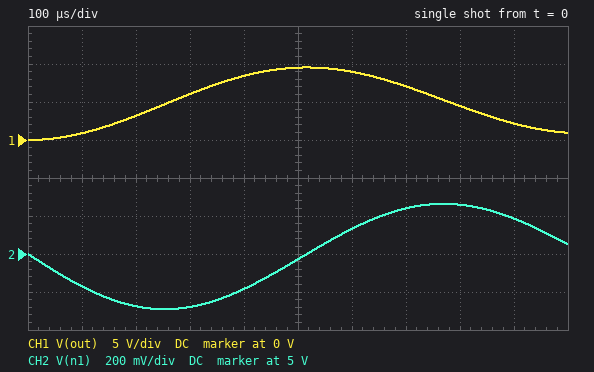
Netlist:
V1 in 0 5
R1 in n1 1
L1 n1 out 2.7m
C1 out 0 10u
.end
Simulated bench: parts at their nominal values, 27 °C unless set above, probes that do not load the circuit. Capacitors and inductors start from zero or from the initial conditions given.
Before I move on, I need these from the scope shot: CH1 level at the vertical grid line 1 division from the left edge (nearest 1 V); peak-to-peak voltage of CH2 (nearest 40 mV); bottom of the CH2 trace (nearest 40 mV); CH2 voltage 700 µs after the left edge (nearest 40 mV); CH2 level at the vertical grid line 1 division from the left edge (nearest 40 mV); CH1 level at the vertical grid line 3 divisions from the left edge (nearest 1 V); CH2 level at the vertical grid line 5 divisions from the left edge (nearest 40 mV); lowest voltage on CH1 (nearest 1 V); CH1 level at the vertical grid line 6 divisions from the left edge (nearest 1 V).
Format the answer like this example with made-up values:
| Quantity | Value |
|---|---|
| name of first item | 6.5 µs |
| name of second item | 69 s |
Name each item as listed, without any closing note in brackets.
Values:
| Quantity | Value |
|---|---|
| CH1 level at the vertical grid line 1 division from the left edge | 1 V |
| peak-to-peak voltage of CH2 | 560 mV |
| bottom of the CH2 trace | 4.72 V |
| CH2 voltage 700 µs after the left edge | 5.24 V |
| CH2 level at the vertical grid line 1 division from the left edge | 4.84 V |
| CH1 level at the vertical grid line 3 divisions from the left edge | 6 V |
| CH2 level at the vertical grid line 5 divisions from the left edge | 4.96 V |
| lowest voltage on CH1 | 0 V |
| CH1 level at the vertical grid line 6 divisions from the left edge | 9 V |
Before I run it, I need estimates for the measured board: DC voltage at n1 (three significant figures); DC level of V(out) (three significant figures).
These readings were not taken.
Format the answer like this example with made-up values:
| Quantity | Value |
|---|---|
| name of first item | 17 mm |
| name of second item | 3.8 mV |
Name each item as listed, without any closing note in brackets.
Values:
| Quantity | Value |
|---|---|
| DC voltage at n1 | 5.00 V |
| DC level of V(out) | 5.00 V |
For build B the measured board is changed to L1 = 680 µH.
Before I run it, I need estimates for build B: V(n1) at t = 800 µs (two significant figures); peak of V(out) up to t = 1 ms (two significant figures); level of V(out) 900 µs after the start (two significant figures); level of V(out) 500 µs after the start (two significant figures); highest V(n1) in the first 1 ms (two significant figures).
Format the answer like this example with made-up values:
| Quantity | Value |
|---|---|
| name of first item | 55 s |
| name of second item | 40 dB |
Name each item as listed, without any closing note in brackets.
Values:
| Quantity | Value |
|---|---|
| V(n1) at t = 800 µs | 5.1 V |
| peak of V(out) up to t = 1 ms | 9.1 V |
| level of V(out) 900 µs after the start | 5.4 V |
| level of V(out) 500 µs after the start | 1.7 V |
| highest V(n1) in the first 1 ms | 5.5 V |
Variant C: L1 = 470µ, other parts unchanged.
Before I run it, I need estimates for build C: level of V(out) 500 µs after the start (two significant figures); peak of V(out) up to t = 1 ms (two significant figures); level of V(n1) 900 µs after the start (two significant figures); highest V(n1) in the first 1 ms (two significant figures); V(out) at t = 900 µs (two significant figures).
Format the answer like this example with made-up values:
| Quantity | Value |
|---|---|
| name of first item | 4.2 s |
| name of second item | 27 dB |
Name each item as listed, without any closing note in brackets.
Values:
| Quantity | Value |
|---|---|
| level of V(out) 500 µs after the start | 3.2 V |
| peak of V(out) up to t = 1 ms | 9.0 V |
| level of V(n1) 900 µs after the start | 4.9 V |
| highest V(n1) in the first 1 ms | 5.5 V |
| V(out) at t = 900 µs | 3.3 V |
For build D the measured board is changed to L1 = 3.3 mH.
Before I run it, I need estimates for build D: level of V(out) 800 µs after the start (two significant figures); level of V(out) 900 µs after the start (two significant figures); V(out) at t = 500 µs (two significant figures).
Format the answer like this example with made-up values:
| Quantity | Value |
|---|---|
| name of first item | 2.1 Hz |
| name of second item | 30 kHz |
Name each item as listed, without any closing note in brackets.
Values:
| Quantity | Value |
|---|---|
| level of V(out) 800 µs after the start | 6.5 V |
| level of V(out) 900 µs after the start | 4.1 V |
| V(out) at t = 500 µs | 9.2 V |
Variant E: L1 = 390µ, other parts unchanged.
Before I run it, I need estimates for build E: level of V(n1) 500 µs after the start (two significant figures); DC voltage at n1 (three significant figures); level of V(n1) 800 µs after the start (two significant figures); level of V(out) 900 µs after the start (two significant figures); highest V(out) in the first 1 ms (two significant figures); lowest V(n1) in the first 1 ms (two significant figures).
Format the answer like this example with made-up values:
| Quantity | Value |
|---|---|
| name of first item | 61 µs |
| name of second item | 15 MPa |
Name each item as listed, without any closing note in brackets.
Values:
| Quantity | Value |
|---|---|
| level of V(n1) 500 µs after the start | 4.6 V |
| DC voltage at n1 | 5.00 V |
| level of V(n1) 800 µs after the start | 4.9 V |
| level of V(out) 900 µs after the start | 5.2 V |
| highest V(out) in the first 1 ms | 8.9 V |
| lowest V(n1) in the first 1 ms | 4.3 V |
